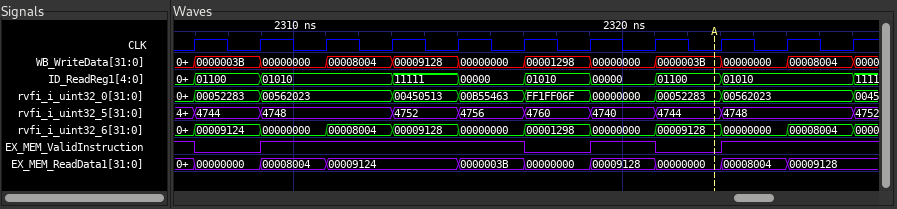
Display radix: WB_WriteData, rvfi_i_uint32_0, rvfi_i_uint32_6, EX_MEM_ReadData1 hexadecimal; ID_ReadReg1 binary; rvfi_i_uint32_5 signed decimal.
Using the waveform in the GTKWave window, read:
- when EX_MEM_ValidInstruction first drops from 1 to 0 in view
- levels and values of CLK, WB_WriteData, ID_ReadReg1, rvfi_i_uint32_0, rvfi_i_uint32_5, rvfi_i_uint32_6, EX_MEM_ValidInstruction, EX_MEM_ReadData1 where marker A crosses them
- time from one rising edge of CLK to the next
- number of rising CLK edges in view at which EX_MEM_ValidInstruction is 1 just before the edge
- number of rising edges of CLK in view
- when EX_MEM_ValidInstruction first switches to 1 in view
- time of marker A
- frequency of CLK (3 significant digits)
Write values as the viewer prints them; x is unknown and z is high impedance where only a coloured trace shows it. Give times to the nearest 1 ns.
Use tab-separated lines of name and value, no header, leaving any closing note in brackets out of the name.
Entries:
when EX_MEM_ValidInstruction first drops from 1 to 0 in view	2307 ns
levels and values of CLK, WB_WriteData, ID_ReadReg1, rvfi_i_uint32_0, rvfi_i_uint32_5, rvfi_i_uint32_6, EX_MEM_ValidInstruction, EX_MEM_ReadData1 where marker A crosses them	CLK=0, WB_WriteData=0000003B, ID_ReadReg1=01100, rvfi_i_uint32_0=00052283, rvfi_i_uint32_5=4744, rvfi_i_uint32_6=00009128, EX_MEM_ValidInstruction=0, EX_MEM_ReadData1=00000000
time from one rising edge of CLK to the next	2 ns
number of rising CLK edges in view at which EX_MEM_ValidInstruction is 1 just before the edge	8
number of rising edges of CLK in view	11
when EX_MEM_ValidInstruction first switches to 1 in view	2309 ns
time of marker A	2323 ns
frequency of CLK	500 MHz
